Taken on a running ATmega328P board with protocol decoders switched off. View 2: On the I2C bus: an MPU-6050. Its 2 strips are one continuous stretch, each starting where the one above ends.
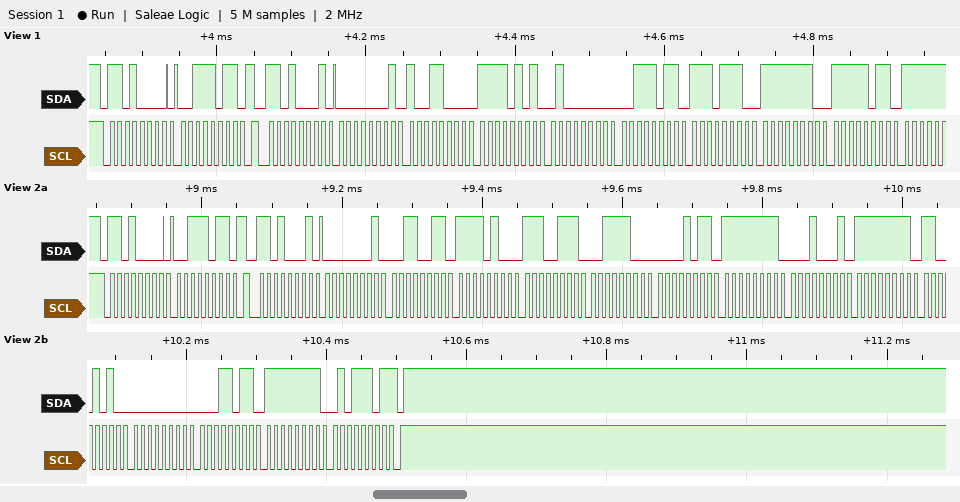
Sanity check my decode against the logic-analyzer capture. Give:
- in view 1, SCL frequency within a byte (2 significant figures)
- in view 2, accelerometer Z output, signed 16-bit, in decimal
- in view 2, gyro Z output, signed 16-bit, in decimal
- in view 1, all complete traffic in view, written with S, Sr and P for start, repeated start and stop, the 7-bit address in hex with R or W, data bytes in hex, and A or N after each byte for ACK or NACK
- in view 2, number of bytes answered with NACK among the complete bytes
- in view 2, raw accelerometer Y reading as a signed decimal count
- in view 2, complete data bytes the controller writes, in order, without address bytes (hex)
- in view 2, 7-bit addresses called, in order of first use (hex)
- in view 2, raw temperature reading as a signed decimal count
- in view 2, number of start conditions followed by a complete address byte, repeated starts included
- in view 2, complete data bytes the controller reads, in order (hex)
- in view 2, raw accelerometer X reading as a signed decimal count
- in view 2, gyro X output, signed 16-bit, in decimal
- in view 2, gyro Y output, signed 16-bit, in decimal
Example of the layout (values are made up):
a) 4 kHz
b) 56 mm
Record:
a) 100 kHz
b) 15371
c) -163
d) S 68W A 3B A Sr 68R A 01 A 98 A F5 A 40 A 3B A EE A FE A FB A
e) 1
f) -2841
g) 3B
h) 0x68
i) -239
j) 2
k) 01 33 F4 E7 3C 0B FF 11 FF CA 00 1B FF 5D
l) 307
m) -54
n) 27
